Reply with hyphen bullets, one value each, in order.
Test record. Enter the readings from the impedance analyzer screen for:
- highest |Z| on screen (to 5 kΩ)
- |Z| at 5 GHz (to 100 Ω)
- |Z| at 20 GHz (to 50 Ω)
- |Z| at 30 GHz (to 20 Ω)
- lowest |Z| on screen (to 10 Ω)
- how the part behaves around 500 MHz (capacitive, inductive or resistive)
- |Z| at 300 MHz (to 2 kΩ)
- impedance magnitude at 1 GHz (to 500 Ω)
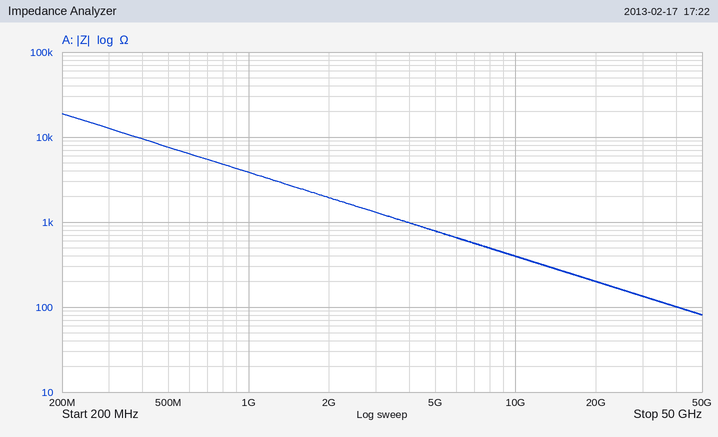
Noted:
- 20 kΩ
- 800 Ω
- 200 Ω
- 140 Ω
- 80 Ω
- capacitive
- 12 kΩ
- 4.0 kΩ
